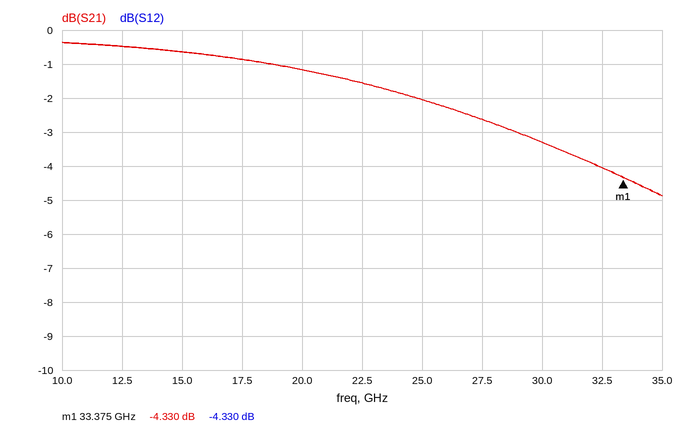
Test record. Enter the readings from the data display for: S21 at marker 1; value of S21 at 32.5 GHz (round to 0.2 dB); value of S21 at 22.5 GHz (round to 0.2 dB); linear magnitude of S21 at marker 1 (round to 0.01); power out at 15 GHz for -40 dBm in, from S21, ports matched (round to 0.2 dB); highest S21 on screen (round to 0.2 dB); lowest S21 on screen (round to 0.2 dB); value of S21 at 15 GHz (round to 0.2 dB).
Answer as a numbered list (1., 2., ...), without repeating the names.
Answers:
1. -4.330 dB
2. -4.0 dB
3. -1.6 dB
4. 0.61
5. -40.6 dBm
6. -0.4 dB
7. -4.8 dB
8. -0.6 dB
